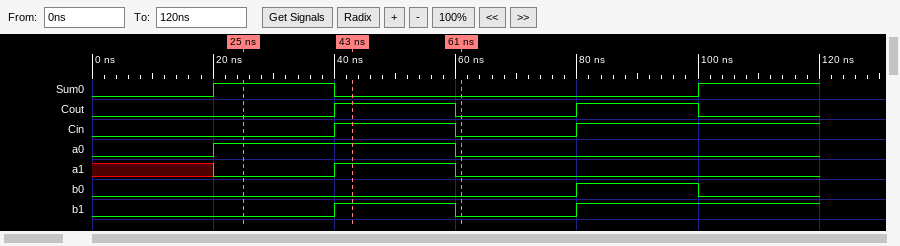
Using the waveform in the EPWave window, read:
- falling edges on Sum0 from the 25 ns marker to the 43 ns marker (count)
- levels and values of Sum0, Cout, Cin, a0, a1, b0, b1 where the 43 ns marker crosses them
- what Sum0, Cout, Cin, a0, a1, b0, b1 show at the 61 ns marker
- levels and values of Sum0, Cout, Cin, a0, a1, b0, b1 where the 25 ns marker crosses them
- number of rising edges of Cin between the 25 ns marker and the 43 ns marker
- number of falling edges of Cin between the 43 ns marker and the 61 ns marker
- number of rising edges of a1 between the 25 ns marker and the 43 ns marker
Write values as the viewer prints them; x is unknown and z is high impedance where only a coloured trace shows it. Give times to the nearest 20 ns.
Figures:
1
Sum0=0, Cout=1, Cin=1, a0=1, a1=1, b0=0, b1=1
Sum0=0, Cout=0, Cin=0, a0=0, a1=0, b0=0, b1=0
Sum0=1, Cout=0, Cin=0, a0=1, a1=0, b0=0, b1=0
1
1
1
